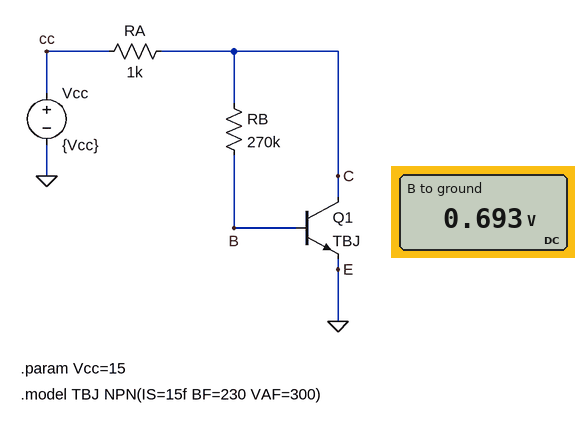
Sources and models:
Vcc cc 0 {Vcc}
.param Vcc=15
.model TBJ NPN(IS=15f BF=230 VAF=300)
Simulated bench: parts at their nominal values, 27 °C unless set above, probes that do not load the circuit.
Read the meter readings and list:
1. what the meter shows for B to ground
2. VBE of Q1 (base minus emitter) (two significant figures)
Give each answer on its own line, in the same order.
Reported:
0.693 V
690 mV
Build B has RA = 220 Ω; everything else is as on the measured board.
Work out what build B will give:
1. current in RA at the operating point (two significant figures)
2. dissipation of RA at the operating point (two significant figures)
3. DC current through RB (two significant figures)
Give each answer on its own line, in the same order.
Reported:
11 mA
25 mW
44 µA
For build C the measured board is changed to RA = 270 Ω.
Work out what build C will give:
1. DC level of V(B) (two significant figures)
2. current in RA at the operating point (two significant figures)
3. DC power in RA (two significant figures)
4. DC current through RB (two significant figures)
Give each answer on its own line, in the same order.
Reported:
700 mV
10 mA
28 mW
43 µA
